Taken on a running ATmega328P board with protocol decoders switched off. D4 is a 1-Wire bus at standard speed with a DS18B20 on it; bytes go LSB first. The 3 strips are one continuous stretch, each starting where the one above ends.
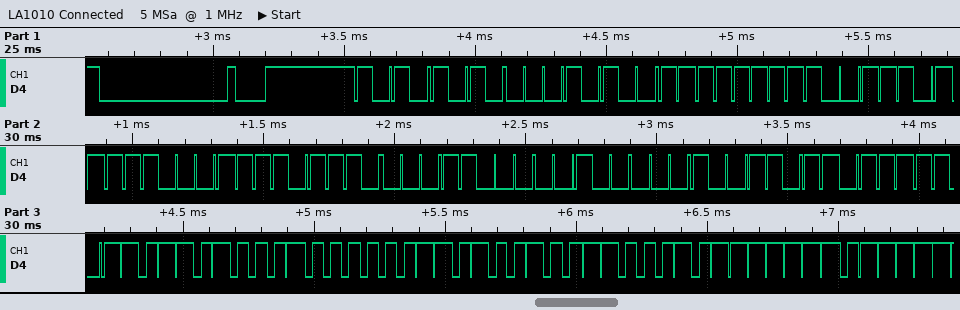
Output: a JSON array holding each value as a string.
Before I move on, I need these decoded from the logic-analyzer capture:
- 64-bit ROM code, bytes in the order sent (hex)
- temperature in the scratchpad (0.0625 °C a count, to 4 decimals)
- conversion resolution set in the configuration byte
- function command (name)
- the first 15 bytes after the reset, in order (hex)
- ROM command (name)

["28 FF B9 8F 77 18 04 D9", "34.8125 °C", "12 bits", "Read Scratchpad", "55 28 FF B9 8F 77 18 04 D9 BE 2D 02 4B 46 7F", "Match ROM"]
